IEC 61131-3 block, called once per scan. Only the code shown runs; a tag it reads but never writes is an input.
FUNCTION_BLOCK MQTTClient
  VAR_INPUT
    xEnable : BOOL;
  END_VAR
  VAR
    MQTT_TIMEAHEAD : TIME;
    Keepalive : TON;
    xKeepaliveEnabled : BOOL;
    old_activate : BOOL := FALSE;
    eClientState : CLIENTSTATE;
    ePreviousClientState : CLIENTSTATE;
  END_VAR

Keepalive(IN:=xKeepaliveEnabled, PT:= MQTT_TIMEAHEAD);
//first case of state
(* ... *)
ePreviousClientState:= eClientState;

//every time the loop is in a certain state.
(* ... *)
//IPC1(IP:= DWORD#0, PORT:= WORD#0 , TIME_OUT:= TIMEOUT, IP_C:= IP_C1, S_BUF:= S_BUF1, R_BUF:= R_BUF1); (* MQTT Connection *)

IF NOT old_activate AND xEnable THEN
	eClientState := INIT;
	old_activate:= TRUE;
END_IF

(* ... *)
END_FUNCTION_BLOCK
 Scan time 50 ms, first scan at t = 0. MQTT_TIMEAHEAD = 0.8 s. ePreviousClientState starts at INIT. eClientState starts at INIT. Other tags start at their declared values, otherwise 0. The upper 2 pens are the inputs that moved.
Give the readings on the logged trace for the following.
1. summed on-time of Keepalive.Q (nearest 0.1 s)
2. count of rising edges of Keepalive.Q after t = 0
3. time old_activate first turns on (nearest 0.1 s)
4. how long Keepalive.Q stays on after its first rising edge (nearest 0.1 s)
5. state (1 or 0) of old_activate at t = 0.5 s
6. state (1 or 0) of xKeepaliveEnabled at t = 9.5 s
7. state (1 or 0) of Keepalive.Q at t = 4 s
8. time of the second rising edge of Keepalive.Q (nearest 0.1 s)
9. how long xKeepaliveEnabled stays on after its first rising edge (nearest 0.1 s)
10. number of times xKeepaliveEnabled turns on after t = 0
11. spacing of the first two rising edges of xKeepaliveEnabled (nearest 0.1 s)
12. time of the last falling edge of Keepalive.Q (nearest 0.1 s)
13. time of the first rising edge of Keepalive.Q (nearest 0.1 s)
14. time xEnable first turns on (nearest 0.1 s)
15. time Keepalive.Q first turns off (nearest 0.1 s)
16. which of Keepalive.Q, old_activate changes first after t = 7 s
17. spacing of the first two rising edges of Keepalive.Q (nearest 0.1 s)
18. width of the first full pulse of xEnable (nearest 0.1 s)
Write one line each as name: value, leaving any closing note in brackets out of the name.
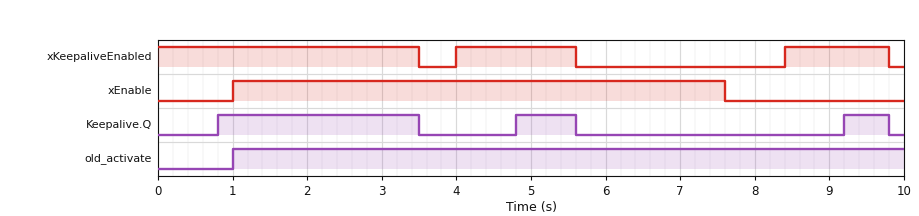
summed on-time of Keepalive.Q: 4.1 s
count of rising edges of Keepalive.Q after t = 0: 3
time old_activate first turns on: 1.0 s
how long Keepalive.Q stays on after its first rising edge: 2.7 s
state (1 or 0) of old_activate at t = 0.5 s: 0
state (1 or 0) of xKeepaliveEnabled at t = 9.5 s: 1
state (1 or 0) of Keepalive.Q at t = 4 s: 0
time of the second rising edge of Keepalive.Q: 4.8 s
how long xKeepaliveEnabled stays on after its first rising edge: 1.6 s
number of times xKeepaliveEnabled turns on after t = 0: 2
spacing of the first two rising edges of xKeepaliveEnabled: 4.4 s
time of the last falling edge of Keepalive.Q: 9.8 s
time of the first rising edge of Keepalive.Q: 0.8 s
time xEnable first turns on: 1.0 s
time Keepalive.Q first turns off: 3.5 s
which of Keepalive.Q, old_activate changes first after t = 7 s: Keepalive.Q
spacing of the first two rising edges of Keepalive.Q: 4.0 s
width of the first full pulse of xEnable: 6.6 s
